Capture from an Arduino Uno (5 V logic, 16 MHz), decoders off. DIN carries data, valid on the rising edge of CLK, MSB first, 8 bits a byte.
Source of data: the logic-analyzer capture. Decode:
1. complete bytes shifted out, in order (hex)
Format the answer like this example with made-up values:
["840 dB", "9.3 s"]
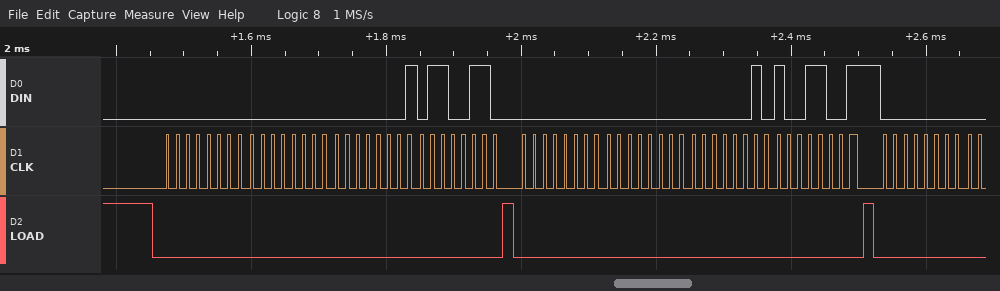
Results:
["00 00 01 66 00 00 02 99 00"]
